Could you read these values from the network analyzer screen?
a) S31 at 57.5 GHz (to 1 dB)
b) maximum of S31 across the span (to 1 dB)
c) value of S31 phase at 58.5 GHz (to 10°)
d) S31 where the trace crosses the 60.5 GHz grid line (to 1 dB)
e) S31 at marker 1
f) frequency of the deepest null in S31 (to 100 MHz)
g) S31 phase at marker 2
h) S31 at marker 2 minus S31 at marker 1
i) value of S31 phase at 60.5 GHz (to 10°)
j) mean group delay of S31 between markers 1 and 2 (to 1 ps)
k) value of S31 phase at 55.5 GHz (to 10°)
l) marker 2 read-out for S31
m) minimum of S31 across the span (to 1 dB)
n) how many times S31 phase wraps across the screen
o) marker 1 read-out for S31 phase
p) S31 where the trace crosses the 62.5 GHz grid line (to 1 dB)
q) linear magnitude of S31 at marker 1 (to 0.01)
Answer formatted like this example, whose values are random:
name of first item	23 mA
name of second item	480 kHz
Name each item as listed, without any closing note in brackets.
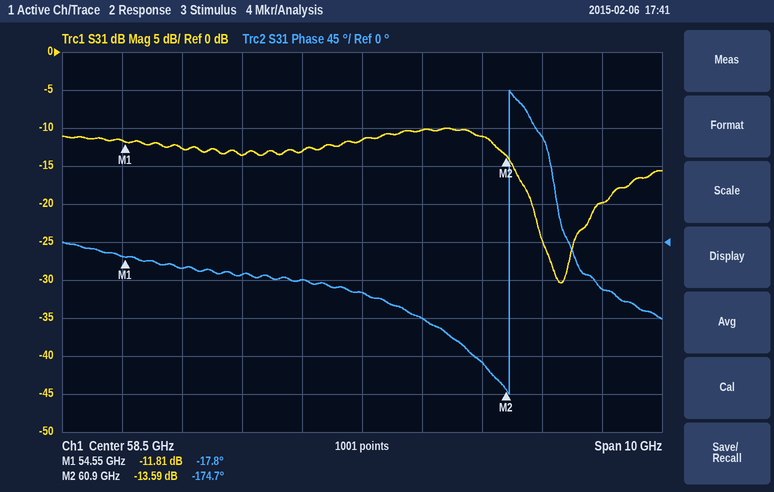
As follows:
S31 at 57.5 GHz	-13 dB
maximum of S31 across the span	-10 dB
value of S31 phase at 58.5 GHz	-60°
S31 where the trace crosses the 60.5 GHz grid line	-11 dB
S31 at marker 1	-11.81 dB
frequency of the deepest null in S31	61.8 GHz
S31 phase at marker 2	-174.7°
S31 at marker 2 minus S31 at marker 1	-1.78 dB
value of S31 phase at 60.5 GHz	-140°
mean group delay of S31 between markers 1 and 2	69 ps
value of S31 phase at 55.5 GHz	-30°
marker 2 read-out for S31	-13.59 dB
minimum of S31 across the span	-30 dB
how many times S31 phase wraps across the screen	1
marker 1 read-out for S31 phase	-17.8°
S31 where the trace crosses the 62.5 GHz grid line	-20 dB
linear magnitude of S31 at marker 1	0.26
